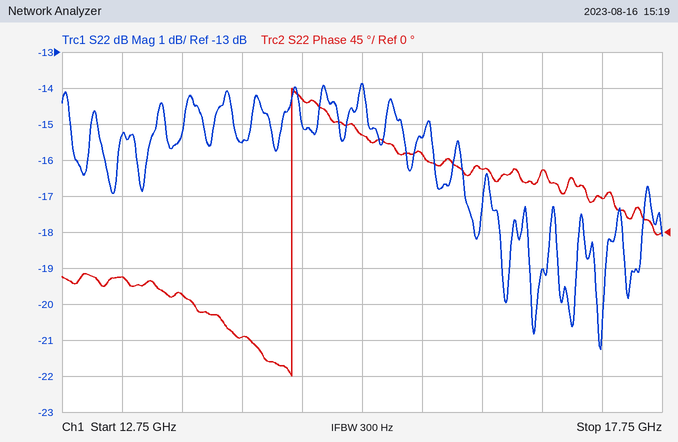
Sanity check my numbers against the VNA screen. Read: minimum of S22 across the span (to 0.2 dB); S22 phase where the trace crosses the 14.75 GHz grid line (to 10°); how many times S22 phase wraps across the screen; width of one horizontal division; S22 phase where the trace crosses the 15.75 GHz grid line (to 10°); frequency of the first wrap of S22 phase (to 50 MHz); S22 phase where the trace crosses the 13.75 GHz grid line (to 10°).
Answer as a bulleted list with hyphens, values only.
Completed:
- -21.2 dB
- 170°
- 1
- 500 MHz
- 100°
- 14.65 GHz
- -80°
